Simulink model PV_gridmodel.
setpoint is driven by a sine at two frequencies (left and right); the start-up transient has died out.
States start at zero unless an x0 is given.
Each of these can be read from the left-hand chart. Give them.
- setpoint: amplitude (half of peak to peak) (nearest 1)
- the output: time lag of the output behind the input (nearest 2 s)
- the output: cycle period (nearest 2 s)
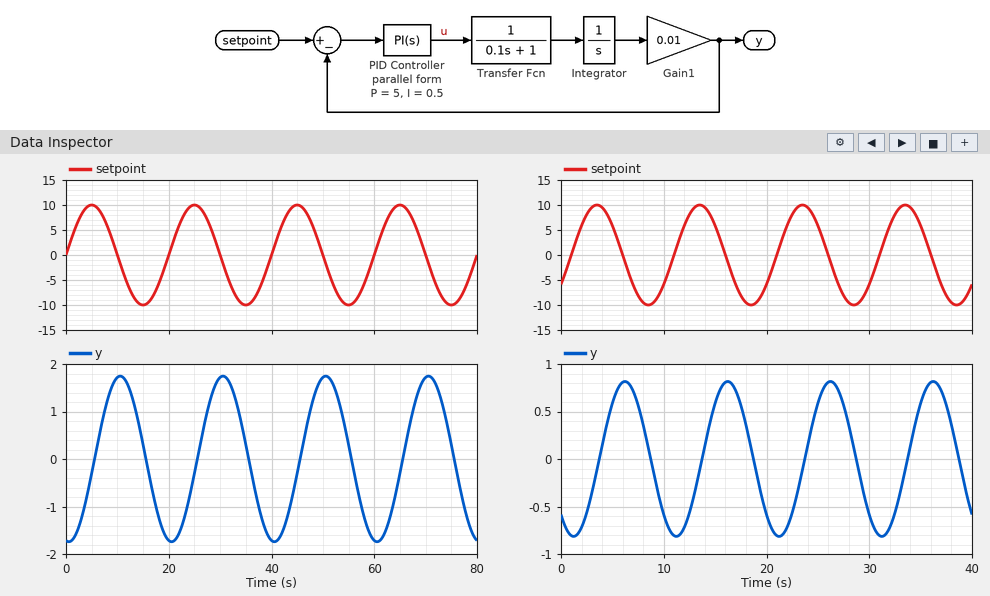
10
6 s
20 s
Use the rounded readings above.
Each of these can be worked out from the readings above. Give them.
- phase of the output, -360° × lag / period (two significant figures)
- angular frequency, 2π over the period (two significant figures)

-110°
0.31 rad/s
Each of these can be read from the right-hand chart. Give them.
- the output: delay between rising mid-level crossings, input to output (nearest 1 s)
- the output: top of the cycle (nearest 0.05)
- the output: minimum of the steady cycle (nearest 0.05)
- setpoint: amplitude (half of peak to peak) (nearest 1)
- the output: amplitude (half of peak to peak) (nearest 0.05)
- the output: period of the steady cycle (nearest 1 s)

3 s
0.80
-0.80
10
0.80
10 s
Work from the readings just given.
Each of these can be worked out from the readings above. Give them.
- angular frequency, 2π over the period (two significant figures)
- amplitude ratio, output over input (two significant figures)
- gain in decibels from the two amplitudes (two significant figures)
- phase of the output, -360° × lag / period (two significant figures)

0.63 rad/s
0.080
-22 dB
-110°
